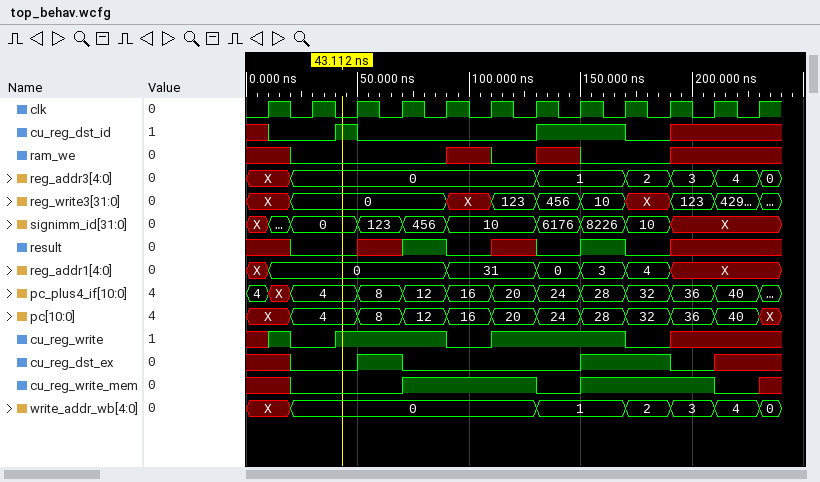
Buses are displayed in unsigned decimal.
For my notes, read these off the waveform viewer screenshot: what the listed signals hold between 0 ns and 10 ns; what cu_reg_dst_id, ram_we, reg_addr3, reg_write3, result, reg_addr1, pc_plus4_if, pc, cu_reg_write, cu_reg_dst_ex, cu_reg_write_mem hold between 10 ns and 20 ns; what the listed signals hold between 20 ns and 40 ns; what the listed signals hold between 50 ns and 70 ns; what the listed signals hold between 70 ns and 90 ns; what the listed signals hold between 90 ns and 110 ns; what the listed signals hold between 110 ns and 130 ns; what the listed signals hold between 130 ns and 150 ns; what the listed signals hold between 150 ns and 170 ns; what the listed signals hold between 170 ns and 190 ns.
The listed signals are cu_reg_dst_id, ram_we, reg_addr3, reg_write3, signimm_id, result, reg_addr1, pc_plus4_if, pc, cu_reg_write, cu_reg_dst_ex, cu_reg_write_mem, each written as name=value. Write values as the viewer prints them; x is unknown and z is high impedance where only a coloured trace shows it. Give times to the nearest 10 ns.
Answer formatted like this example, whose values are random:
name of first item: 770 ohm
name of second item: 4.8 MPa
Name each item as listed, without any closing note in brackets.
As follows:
what the listed signals hold between 0 ns and 10 ns: cu_reg_dst_id=x, ram_we=x, reg_addr3=X, reg_write3=X, signimm_id=X, result=x, reg_addr1=X, pc_plus4_if=4, pc=X, cu_reg_write=x, cu_reg_dst_ex=x, cu_reg_write_mem=x
what cu_reg_dst_id, ram_we, reg_addr3, reg_write3, result, reg_addr1, pc_plus4_if, pc, cu_reg_write, cu_reg_dst_ex, cu_reg_write_mem hold between 10 ns and 20 ns: cu_reg_dst_id=0, ram_we=x, reg_addr3=X, reg_write3=X, result=x, reg_addr1=0, pc_plus4_if=X, pc=X, cu_reg_write=1, cu_reg_dst_ex=x, cu_reg_write_mem=x
what the listed signals hold between 20 ns and 40 ns: cu_reg_dst_id=0, ram_we=0, reg_addr3=0, reg_write3=0, signimm_id=0, result=0, reg_addr1=0, pc_plus4_if=4, pc=4, cu_reg_write=0, cu_reg_dst_ex=0, cu_reg_write_mem=0
what the listed signals hold between 50 ns and 70 ns: cu_reg_dst_id=0, ram_we=0, reg_addr3=0, reg_write3=0, signimm_id=123, result=x, reg_addr1=0, pc_plus4_if=8, pc=8, cu_reg_write=1, cu_reg_dst_ex=1, cu_reg_write_mem=0
what the listed signals hold between 70 ns and 90 ns: cu_reg_dst_id=0, ram_we=0, reg_addr3=0, reg_write3=0, signimm_id=456, result=1, reg_addr1=0, pc_plus4_if=12, pc=12, cu_reg_write=1, cu_reg_dst_ex=0, cu_reg_write_mem=1
what the listed signals hold between 90 ns and 110 ns: cu_reg_dst_id=0, ram_we=x, reg_addr3=0, reg_write3=X, signimm_id=10, result=0, reg_addr1=31, pc_plus4_if=16, pc=16, cu_reg_write=0, cu_reg_dst_ex=0, cu_reg_write_mem=1
what the listed signals hold between 110 ns and 130 ns: cu_reg_dst_id=0, ram_we=0, reg_addr3=0, reg_write3=123, signimm_id=10, result=x, reg_addr1=31, pc_plus4_if=20, pc=20, cu_reg_write=1, cu_reg_dst_ex=0, cu_reg_write_mem=1
what the listed signals hold between 130 ns and 150 ns: cu_reg_dst_id=1, ram_we=x, reg_addr3=1, reg_write3=456, signimm_id=6176, result=0, reg_addr1=0, pc_plus4_if=24, pc=24, cu_reg_write=1, cu_reg_dst_ex=0, cu_reg_write_mem=0
what the listed signals hold between 150 ns and 170 ns: cu_reg_dst_id=1, ram_we=0, reg_addr3=1, reg_write3=10, signimm_id=8226, result=1, reg_addr1=3, pc_plus4_if=28, pc=28, cu_reg_write=1, cu_reg_dst_ex=1, cu_reg_write_mem=1
what the listed signals hold between 170 ns and 190 ns: cu_reg_dst_id=0, ram_we=0, reg_addr3=2, reg_write3=X, signimm_id=10, result=0, reg_addr1=4, pc_plus4_if=32, pc=32, cu_reg_write=0, cu_reg_dst_ex=1, cu_reg_write_mem=1
